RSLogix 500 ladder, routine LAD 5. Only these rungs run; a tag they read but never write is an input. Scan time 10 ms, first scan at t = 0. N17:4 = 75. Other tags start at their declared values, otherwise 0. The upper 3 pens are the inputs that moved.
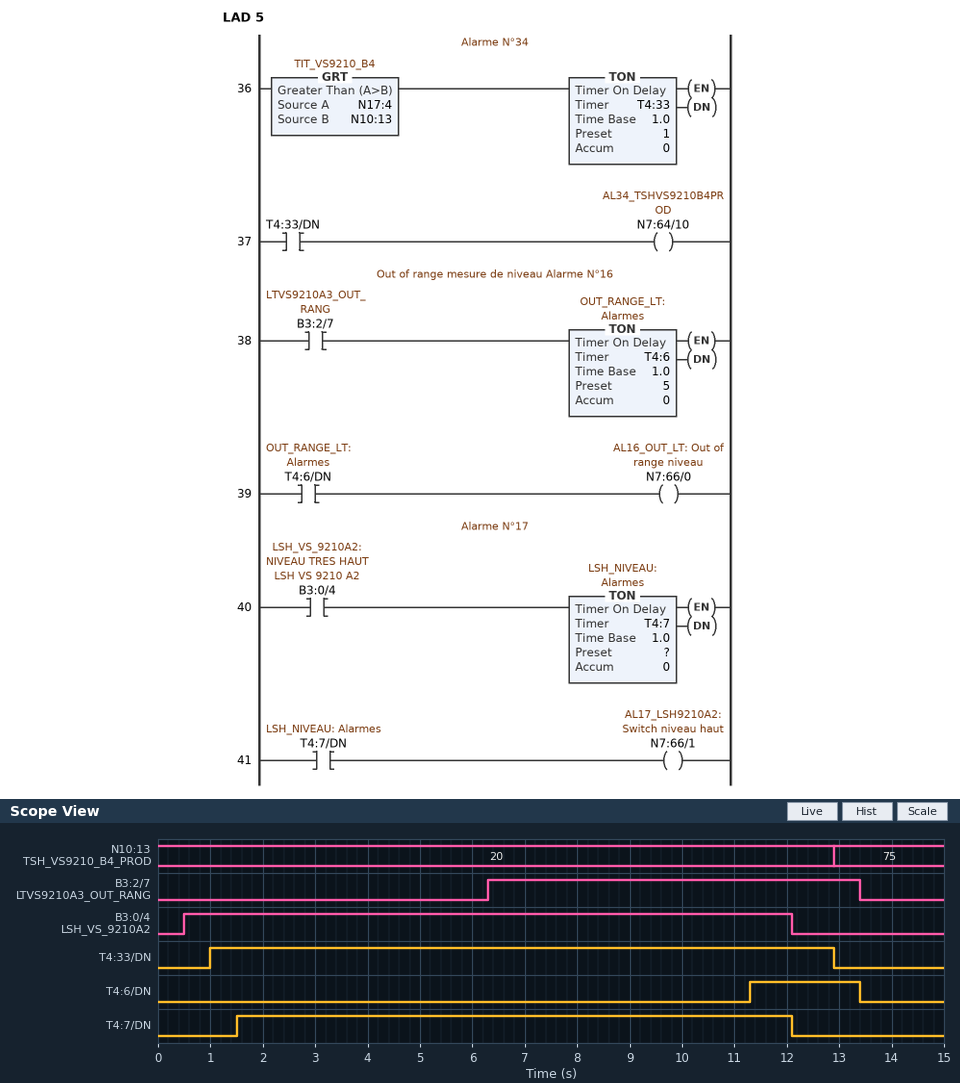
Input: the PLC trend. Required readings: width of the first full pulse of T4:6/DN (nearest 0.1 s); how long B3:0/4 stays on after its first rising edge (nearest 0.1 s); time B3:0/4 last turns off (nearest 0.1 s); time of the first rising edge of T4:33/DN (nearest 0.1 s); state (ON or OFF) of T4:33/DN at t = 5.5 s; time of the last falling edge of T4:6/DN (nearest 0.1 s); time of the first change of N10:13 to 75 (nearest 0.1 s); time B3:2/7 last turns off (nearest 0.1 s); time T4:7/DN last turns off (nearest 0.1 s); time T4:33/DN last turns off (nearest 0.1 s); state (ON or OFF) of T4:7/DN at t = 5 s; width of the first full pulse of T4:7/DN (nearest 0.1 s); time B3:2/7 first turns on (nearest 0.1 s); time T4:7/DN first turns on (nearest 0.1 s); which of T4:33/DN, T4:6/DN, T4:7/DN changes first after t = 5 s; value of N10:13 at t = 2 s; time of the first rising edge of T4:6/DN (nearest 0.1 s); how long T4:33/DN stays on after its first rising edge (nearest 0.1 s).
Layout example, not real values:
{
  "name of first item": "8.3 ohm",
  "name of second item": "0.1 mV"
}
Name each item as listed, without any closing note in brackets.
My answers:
{
  "width of the first full pulse of T4:6/DN": "2.1 s",
  "how long B3:0/4 stays on after its first rising edge": "11.6 s",
  "time B3:0/4 last turns off": "12.1 s",
  "time of the first rising edge of T4:33/DN": "1.0 s",
  "state (ON or OFF) of T4:33/DN at t = 5.5 s": "ON",
  "time of the last falling edge of T4:6/DN": "13.4 s",
  "time of the first change of N10:13 to 75": "12.9 s",
  "time B3:2/7 last turns off": "13.4 s",
  "time T4:7/DN last turns off": "12.1 s",
  "time T4:33/DN last turns off": "12.9 s",
  "state (ON or OFF) of T4:7/DN at t = 5 s": "ON",
  "width of the first full pulse of T4:7/DN": "10.6 s",
  "time B3:2/7 first turns on": "6.3 s",
  "time T4:7/DN first turns on": "1.5 s",
  "which of T4:33/DN, T4:6/DN, T4:7/DN changes first after t = 5 s": "T4:6/DN",
  "value of N10:13 at t = 2 s": "20",
  "time of the first rising edge of T4:6/DN": "11.3 s",
  "how long T4:33/DN stays on after its first rising edge": "11.9 s"
}
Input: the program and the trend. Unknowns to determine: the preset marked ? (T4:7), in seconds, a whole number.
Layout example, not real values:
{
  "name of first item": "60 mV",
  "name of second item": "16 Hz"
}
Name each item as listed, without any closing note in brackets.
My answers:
{
  "the preset marked ? (T4:7), in seconds, a whole number": "1 s"
}
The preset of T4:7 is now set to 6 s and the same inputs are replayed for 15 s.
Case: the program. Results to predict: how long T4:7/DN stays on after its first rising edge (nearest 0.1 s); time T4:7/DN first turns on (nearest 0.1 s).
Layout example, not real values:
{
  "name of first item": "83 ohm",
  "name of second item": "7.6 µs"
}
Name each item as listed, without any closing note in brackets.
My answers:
{
  "how long T4:7/DN stays on after its first rising edge": "5.6 s",
  "time T4:7/DN first turns on": "6.5 s"
}
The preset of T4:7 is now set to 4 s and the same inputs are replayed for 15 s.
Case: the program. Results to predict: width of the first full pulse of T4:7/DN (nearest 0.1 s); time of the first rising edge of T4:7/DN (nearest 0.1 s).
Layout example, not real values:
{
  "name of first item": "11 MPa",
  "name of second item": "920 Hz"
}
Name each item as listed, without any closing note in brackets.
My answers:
{
  "width of the first full pulse of T4:7/DN": "7.6 s",
  "time of the first rising edge of T4:7/DN": "4.5 s"
}
